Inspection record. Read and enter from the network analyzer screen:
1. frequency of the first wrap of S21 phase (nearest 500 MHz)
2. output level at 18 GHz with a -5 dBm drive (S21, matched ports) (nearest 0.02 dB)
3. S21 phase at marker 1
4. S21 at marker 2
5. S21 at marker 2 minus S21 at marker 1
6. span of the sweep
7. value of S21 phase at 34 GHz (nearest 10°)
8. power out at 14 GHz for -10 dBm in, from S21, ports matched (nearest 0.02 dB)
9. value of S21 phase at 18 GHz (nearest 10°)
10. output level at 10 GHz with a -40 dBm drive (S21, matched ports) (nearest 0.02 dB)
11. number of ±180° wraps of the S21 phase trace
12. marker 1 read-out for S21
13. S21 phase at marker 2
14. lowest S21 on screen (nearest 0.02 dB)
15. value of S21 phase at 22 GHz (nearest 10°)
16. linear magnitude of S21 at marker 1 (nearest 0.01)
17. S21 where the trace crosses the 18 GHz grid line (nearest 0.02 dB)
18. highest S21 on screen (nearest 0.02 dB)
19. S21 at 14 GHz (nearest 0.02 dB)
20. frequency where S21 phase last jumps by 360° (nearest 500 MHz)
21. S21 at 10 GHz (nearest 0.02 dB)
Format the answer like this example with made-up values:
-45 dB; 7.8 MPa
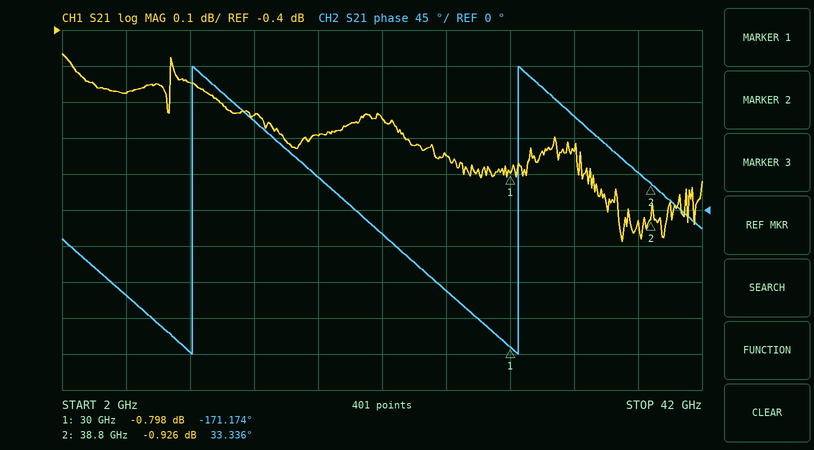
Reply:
10.0 GHz; -5.70 dBm; -171.174°; -0.926 dB; -0.128 dB; 40 GHz; 120°; -10.64 dBm; 40°; -40.54 dBm; 2; -0.798 dB; 33.336°; -0.98 dB; -30°; 0.91; -0.70 dB; -0.46 dB; -0.64 dB; 30.5 GHz; -0.54 dB
